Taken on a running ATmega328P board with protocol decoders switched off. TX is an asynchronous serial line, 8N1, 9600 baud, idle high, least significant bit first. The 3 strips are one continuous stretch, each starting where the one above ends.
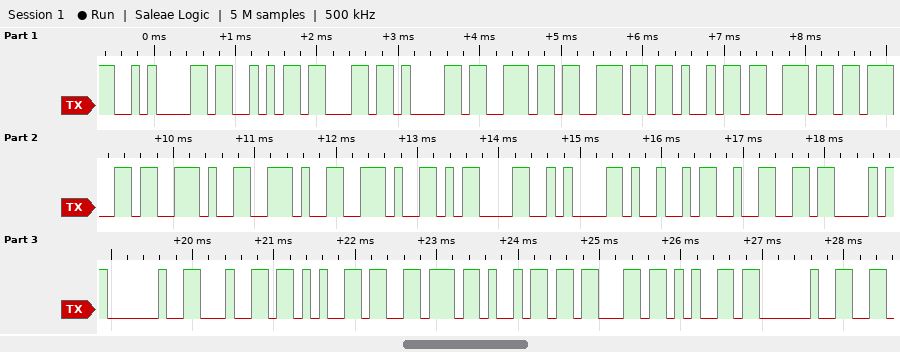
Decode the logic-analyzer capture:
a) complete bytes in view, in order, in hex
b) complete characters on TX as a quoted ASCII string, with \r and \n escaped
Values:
0A 53 63 61 6E 6E 69 6E 67 2E 2E 2E 0D 0A 49 32 43 20 64 65 76 69 63 65 20
"\nScanning...\r\nI2C device "
